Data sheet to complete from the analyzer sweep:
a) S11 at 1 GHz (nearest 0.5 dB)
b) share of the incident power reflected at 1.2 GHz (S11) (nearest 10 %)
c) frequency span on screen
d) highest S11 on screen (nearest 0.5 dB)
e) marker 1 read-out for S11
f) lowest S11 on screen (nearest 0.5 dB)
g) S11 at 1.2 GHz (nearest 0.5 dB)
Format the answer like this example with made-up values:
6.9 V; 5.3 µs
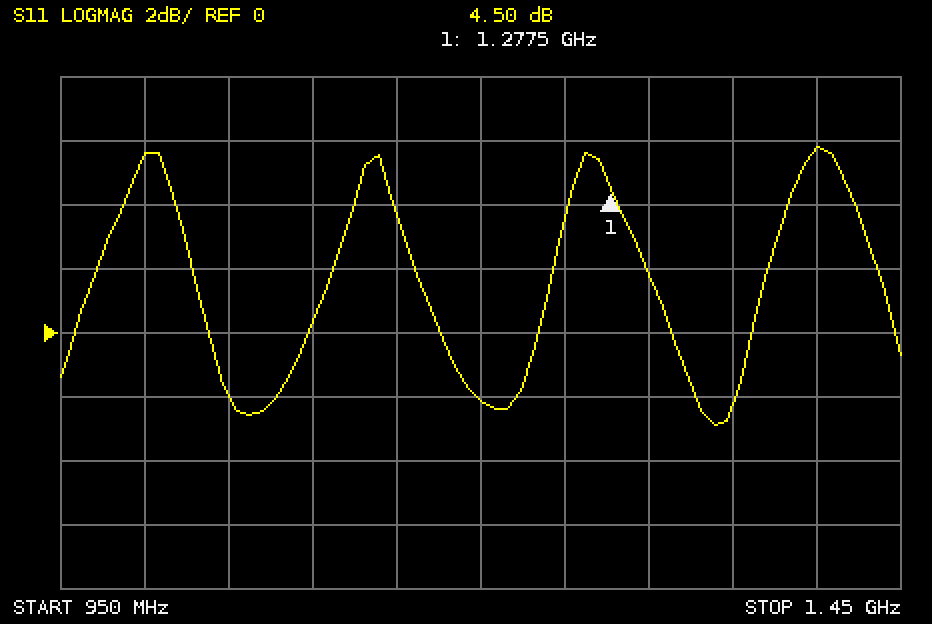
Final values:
5.5 dB; 60 %; 500 MHz; 6.0 dB; 4.50 dB; -3.0 dB; -2.0 dB
